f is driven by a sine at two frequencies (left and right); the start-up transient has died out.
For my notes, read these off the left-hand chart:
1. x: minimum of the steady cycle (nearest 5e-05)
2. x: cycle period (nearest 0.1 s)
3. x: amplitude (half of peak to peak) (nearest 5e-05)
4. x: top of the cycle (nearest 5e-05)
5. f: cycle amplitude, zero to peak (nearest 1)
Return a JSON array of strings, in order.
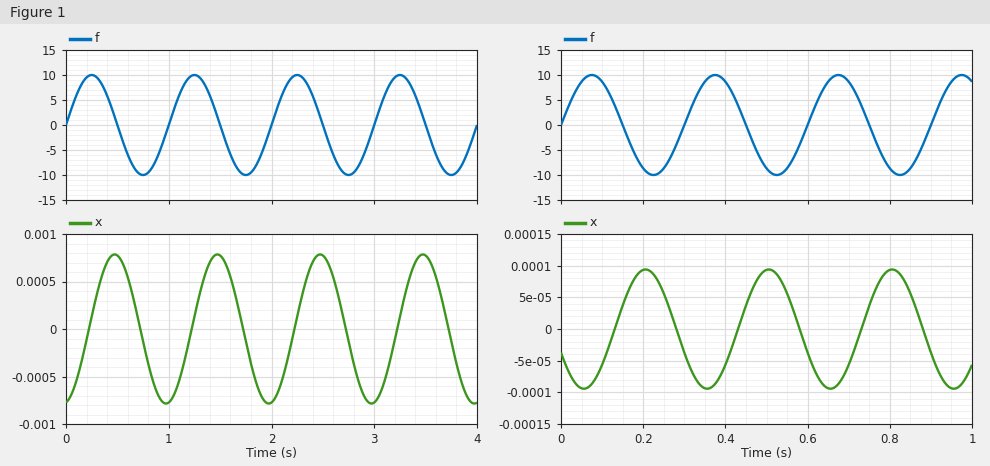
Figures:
["-0.00080", "1.0 s", "0.00080", "0.00080", "10"]
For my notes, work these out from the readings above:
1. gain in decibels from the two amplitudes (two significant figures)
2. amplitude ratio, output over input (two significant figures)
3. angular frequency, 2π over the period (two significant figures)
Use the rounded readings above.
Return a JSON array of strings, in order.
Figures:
["-82 dB", "0.000080", "6.3 rad/s"]
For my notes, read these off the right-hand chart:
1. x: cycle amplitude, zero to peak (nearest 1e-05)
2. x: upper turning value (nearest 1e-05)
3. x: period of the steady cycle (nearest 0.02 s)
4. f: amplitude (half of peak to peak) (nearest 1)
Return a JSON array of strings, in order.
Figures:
["0.00009", "0.00009", "0.30 s", "10"]
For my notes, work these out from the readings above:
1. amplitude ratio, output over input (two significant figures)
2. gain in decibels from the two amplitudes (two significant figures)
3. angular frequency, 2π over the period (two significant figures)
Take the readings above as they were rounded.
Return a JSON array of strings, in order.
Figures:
["0.0000090", "-100 dB", "21 rad/s"]
